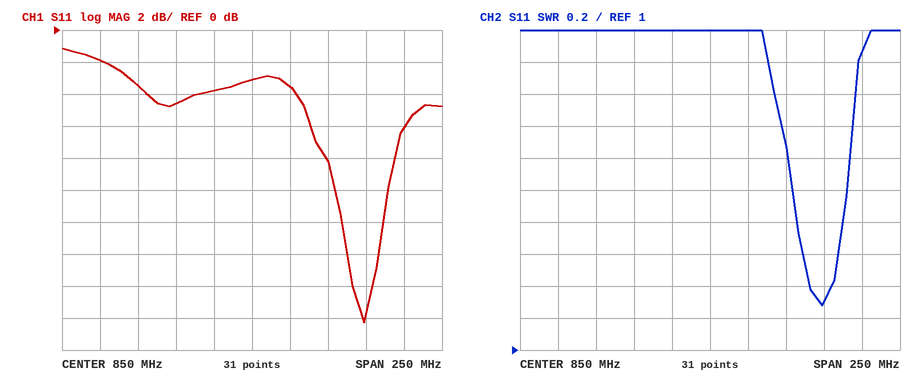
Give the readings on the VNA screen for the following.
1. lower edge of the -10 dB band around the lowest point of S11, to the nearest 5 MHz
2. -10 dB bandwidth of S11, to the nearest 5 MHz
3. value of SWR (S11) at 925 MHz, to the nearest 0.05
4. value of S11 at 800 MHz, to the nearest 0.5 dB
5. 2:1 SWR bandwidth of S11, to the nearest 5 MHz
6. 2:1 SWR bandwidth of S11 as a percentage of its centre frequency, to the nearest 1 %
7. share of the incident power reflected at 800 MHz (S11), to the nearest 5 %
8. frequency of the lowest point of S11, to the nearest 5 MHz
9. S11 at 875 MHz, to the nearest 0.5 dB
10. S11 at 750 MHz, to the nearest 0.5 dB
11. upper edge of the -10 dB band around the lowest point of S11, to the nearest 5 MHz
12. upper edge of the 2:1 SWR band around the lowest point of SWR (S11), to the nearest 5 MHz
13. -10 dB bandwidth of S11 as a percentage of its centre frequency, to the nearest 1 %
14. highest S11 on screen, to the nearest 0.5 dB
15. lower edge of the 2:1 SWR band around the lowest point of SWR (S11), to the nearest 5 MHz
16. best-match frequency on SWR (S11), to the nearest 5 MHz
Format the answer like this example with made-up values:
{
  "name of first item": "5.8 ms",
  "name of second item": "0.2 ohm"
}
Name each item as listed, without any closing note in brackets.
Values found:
{
  "lower edge of the -10 dB band around the lowest point of S11, to the nearest 5 MHz": "905 MHz",
  "-10 dB bandwidth of S11, to the nearest 5 MHz": "35 MHz",
  "value of SWR (S11) at 925 MHz, to the nearest 0.05": "1.30",
  "value of S11 at 800 MHz, to the nearest 0.5 dB": "-4.5 dB",
  "2:1 SWR bandwidth of S11, to the nearest 5 MHz": "35 MHz",
  "2:1 SWR bandwidth of S11 as a percentage of its centre frequency, to the nearest 1 %": "4 %",
  "share of the incident power reflected at 800 MHz (S11), to the nearest 5 %": "35 %",
  "frequency of the lowest point of S11, to the nearest 5 MHz": "925 MHz",
  "S11 at 875 MHz, to the nearest 0.5 dB": "-3.5 dB",
  "S11 at 750 MHz, to the nearest 0.5 dB": "-2.0 dB",
  "upper edge of the -10 dB band around the lowest point of S11, to the nearest 5 MHz": "940 MHz",
  "upper edge of the 2:1 SWR band around the lowest point of SWR (S11), to the nearest 5 MHz": "940 MHz",
  "-10 dB bandwidth of S11 as a percentage of its centre frequency, to the nearest 1 %": "4 %",
  "highest S11 on screen, to the nearest 0.5 dB": "-1.0 dB",
  "lower edge of the 2:1 SWR band around the lowest point of SWR (S11), to the nearest 5 MHz": "905 MHz",
  "best-match frequency on SWR (S11), to the nearest 5 MHz": "925 MHz"
}
